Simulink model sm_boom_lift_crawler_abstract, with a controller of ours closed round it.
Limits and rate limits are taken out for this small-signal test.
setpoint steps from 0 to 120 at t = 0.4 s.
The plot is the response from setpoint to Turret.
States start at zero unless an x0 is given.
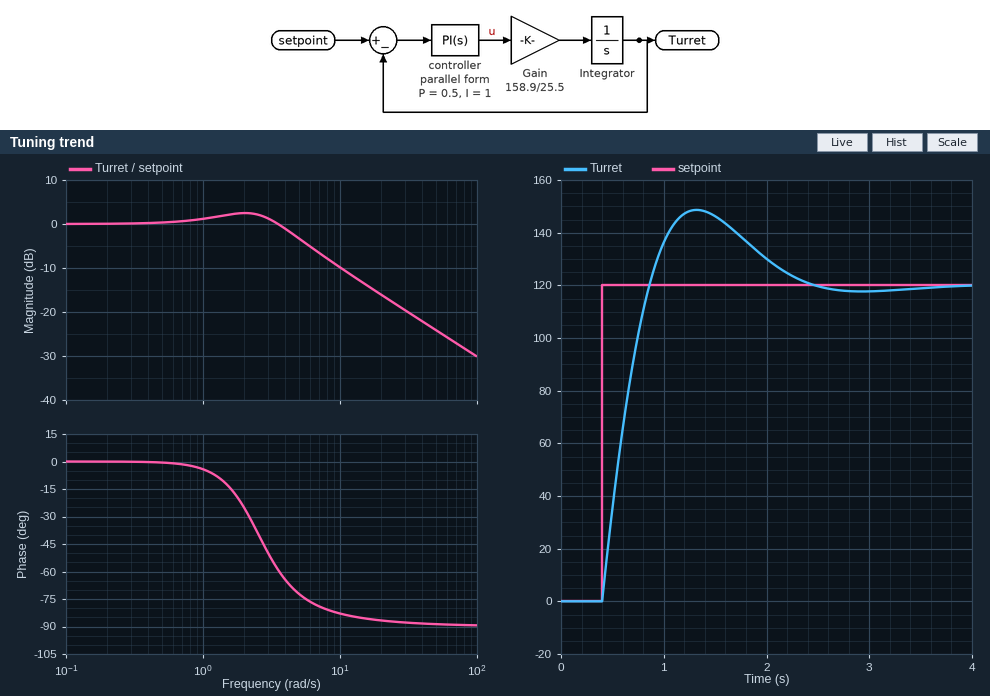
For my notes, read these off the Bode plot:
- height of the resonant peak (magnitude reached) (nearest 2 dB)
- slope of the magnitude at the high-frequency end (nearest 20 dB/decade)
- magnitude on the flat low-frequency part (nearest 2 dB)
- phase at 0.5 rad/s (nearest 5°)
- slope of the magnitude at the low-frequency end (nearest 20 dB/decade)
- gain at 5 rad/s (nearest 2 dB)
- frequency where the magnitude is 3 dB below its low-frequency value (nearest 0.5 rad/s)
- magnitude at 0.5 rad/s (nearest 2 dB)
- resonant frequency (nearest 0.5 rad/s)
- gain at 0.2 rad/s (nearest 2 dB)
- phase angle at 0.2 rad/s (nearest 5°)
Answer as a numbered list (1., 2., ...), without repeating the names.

1. 2 dB
2. -20 dB/decade
3. 0 dB
4. 0°
5. 0 dB/decade
6. -4 dB
7. 5.0 rad/s
8. 0 dB
9. 2.0 rad/s
10. 0 dB
11. 0°
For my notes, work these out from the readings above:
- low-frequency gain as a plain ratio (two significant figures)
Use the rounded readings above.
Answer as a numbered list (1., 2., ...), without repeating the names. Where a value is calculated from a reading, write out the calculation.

1. 10^(0 / 20) = 1.0
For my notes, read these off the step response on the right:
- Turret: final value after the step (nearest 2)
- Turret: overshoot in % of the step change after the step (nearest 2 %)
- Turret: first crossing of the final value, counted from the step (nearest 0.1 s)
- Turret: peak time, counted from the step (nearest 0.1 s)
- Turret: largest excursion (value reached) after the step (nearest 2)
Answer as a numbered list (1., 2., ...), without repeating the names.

1. 120
2. 24 %
3. 0.5 s
4. 0.9 s
5. 148
